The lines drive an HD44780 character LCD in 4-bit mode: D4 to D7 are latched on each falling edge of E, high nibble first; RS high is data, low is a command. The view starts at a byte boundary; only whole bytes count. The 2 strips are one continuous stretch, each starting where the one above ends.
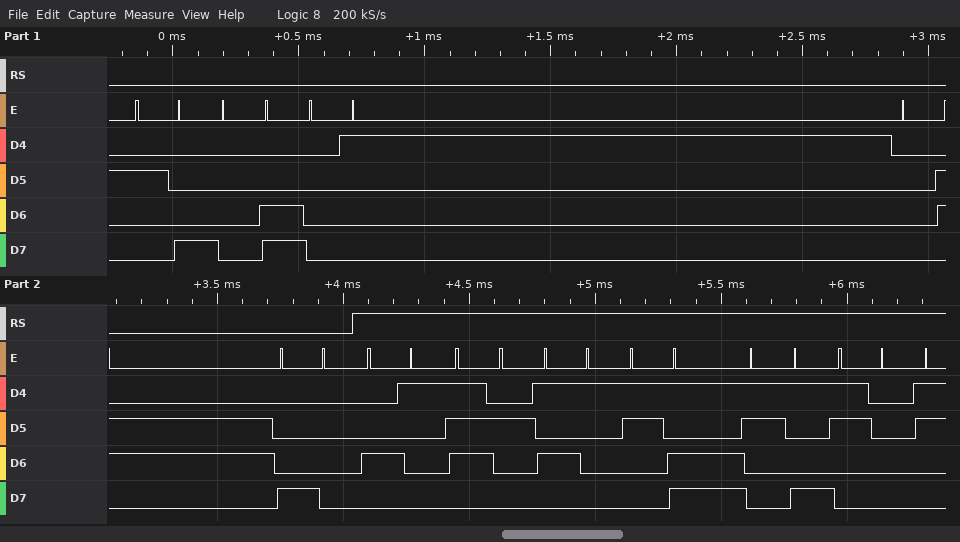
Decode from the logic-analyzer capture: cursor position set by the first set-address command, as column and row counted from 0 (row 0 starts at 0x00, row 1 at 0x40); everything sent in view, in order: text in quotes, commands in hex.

column 0, row 0
0x28 0x0C 0x01 0x06 0x80 "ArQ=90"
